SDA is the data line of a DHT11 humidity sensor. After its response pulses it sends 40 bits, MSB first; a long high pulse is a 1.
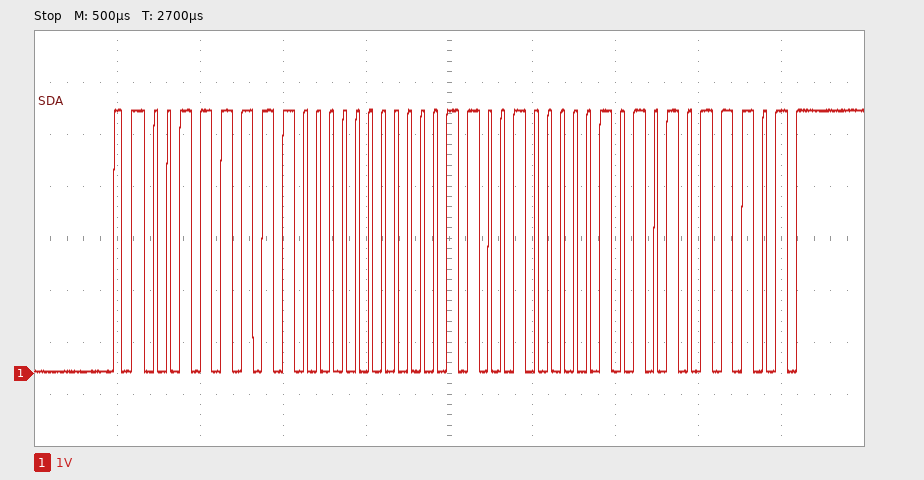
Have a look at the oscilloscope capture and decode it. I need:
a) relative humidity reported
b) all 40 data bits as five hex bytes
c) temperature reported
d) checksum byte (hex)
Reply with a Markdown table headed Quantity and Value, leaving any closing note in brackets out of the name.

| Quantity | Value |
|---|---|
| relative humidity reported | 63 % |
| all 40 data bits as five hex bytes | 3F 00 19 05 5D |
| temperature reported | 25.5 °C |
| checksum byte | 0x5D |
